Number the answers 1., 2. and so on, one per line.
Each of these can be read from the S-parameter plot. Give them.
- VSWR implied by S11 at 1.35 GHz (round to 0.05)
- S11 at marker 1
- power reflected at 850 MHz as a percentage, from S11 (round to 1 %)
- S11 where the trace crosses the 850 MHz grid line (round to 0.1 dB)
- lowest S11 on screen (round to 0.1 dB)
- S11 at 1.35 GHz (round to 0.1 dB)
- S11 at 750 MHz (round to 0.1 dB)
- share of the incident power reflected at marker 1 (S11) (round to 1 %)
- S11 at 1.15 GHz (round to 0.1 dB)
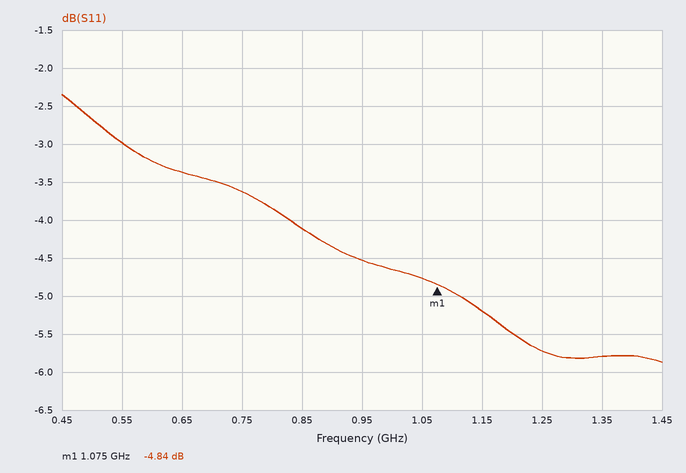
1. 3.10
2. -4.84 dB
3. 39 %
4. -4.1 dB
5. -5.9 dB
6. -5.8 dB
7. -3.6 dB
8. 33 %
9. -5.2 dB
